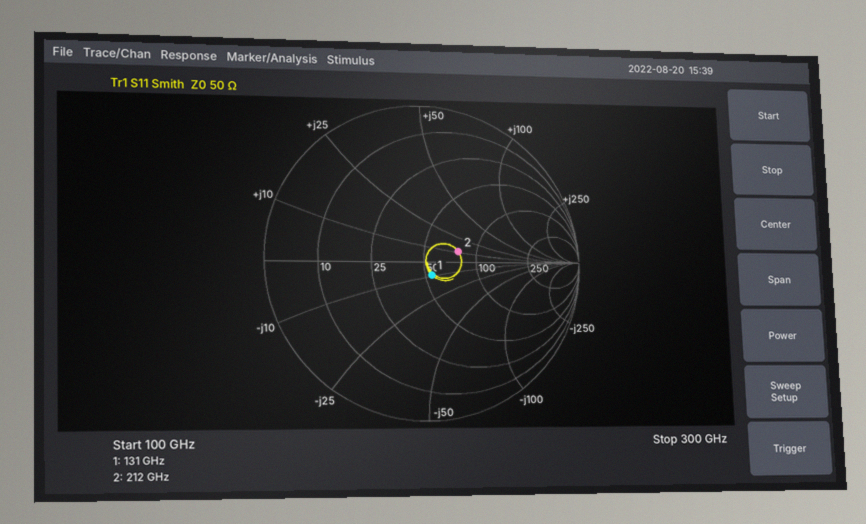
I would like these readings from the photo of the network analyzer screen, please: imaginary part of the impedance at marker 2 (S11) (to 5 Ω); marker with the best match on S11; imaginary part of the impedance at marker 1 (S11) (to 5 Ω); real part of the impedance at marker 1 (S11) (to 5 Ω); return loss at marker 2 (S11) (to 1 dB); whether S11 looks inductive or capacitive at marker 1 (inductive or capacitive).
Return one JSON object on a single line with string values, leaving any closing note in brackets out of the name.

{"imaginary part of the impedance at marker 2 (S11)": "+10 Ω", "marker with the best match on S11": "marker 1", "imaginary part of the impedance at marker 1 (S11)": "-10 Ω", "real part of the impedance at marker 1 (S11)": "55 Ω", "return loss at marker 2 (S11)": "13 dB", "whether S11 looks inductive or capacitive at marker 1": "capacitive"}
